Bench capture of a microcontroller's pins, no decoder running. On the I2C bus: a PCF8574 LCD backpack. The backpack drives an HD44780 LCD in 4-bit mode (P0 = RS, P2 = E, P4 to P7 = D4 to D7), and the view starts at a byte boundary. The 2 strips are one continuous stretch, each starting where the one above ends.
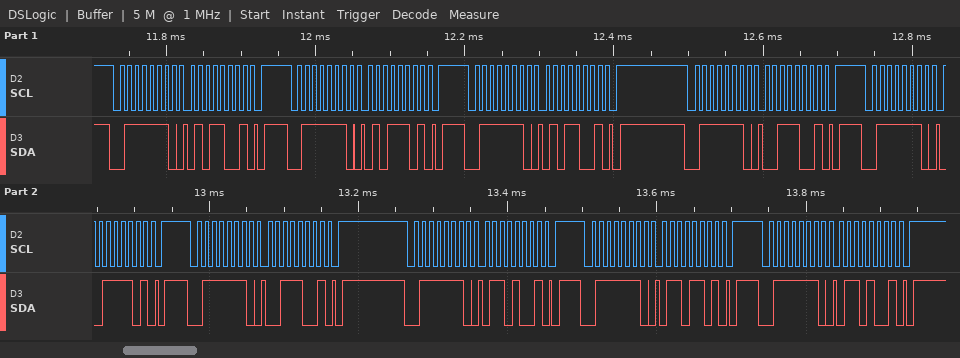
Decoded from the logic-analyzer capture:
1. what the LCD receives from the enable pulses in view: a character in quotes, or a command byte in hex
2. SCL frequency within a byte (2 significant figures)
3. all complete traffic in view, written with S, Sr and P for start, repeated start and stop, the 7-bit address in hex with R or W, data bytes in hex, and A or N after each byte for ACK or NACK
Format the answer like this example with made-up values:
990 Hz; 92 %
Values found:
'S'; 100 kHz; S 3FW A 59 A P S 3FW A 5D A P S 3FW A 59 A P S 3FW A 39 A P S 3FW A 3D A P S 3FW A 39 A P S 3FW A 69 A P S 3FW A 6D A P S 3FW A 69 A P
